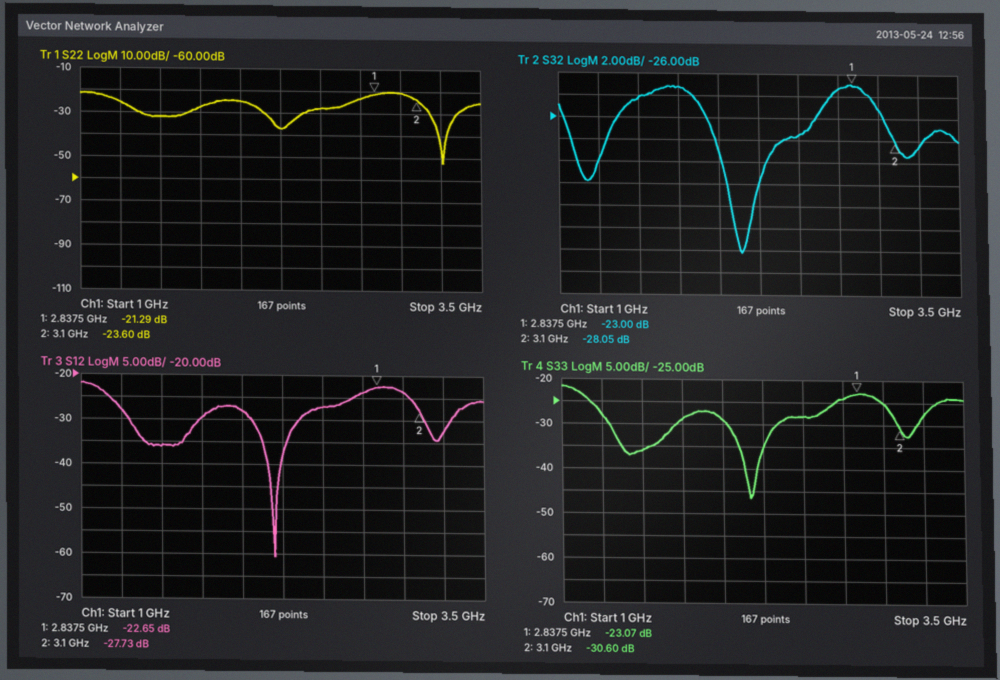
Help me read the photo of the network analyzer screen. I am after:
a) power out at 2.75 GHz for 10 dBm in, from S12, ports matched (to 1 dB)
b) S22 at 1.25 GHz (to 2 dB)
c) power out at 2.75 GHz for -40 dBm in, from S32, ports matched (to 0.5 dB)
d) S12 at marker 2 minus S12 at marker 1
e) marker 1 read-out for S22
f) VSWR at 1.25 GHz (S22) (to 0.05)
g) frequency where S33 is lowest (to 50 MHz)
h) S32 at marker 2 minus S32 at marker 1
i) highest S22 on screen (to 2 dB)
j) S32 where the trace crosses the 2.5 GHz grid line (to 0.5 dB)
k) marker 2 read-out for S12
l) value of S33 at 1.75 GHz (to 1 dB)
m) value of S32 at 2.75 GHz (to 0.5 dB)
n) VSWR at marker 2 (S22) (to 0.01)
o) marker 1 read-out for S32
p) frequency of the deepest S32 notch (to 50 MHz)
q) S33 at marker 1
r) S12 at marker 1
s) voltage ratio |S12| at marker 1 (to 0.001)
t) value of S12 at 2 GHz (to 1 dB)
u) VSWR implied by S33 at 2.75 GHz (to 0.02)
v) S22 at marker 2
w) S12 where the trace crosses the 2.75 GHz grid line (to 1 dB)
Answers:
-14 dBm
-26 dB
-63.5 dBm
-5.08 dB
-21.29 dB
1.10
2.15 GHz
-5.05 dB
-20 dB
-27.5 dB
-27.73 dB
-29 dB
-23.5 dB
1.14
-23.00 dB
2.15 GHz
-23.07 dB
-22.65 dB
0.074
-28 dB
1.14
-23.60 dB
-24 dB
